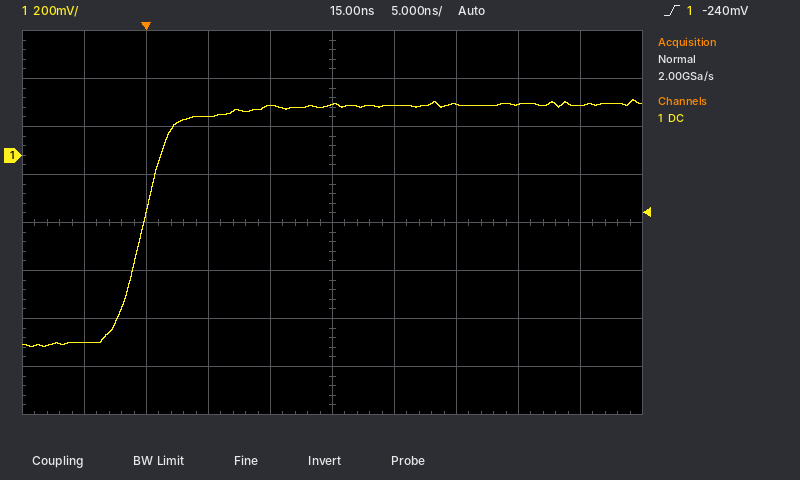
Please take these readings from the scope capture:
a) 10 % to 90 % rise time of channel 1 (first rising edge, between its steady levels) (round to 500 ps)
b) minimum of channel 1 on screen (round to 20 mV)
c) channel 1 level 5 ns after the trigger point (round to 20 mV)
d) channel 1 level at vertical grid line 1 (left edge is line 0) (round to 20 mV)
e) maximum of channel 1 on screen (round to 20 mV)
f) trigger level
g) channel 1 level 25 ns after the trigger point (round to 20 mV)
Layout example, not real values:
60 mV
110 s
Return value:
4.5 ns
-800 mV
160 mV
-780 mV
240 mV
-240 mV
220 mV
